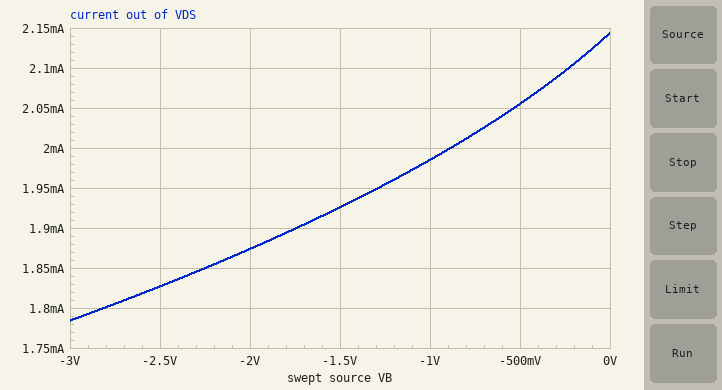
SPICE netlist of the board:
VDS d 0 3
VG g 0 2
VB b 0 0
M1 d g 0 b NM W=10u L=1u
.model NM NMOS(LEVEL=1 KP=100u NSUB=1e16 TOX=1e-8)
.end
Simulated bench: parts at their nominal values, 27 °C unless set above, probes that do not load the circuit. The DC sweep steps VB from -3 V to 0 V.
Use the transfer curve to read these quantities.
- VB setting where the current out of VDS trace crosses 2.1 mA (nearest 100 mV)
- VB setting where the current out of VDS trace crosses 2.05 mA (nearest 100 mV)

-200 mV
-500 mV
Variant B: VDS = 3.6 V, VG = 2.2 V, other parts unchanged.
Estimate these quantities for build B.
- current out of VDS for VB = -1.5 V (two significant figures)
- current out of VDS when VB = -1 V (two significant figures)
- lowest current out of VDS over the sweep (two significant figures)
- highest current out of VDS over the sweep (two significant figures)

2.3 mA
2.4 mA
2.2 mA
2.6 mA
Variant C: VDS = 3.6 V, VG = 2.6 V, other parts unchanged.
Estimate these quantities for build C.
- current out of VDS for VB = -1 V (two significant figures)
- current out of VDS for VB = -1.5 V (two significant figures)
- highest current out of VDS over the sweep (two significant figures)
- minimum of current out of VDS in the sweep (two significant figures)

3.4 mA
3.3 mA
3.6 mA
3.1 mA
